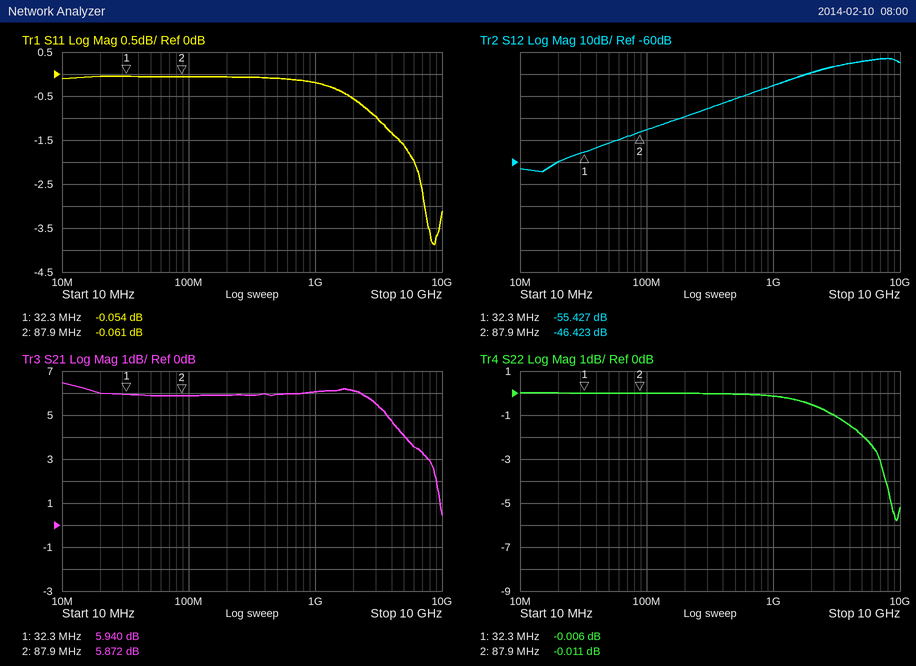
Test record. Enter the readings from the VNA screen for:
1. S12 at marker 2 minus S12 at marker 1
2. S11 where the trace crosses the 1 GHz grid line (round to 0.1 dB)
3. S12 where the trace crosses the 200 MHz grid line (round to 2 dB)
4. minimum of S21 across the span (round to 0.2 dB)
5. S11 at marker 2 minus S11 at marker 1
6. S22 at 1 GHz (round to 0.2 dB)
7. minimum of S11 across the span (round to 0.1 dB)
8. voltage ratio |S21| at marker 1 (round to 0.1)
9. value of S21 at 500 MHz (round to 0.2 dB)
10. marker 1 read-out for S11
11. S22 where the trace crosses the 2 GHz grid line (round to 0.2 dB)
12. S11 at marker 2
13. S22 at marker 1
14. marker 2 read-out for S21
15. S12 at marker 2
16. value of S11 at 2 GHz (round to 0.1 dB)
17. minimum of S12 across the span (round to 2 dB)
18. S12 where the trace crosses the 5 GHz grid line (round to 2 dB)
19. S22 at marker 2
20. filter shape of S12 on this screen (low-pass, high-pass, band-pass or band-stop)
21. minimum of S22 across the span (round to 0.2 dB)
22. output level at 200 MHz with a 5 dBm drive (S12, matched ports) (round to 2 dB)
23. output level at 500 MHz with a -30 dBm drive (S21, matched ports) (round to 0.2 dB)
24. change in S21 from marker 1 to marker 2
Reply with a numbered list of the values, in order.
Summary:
1. 9.004 dB
2. -0.2 dB
3. -40 dB
4. 0.4 dB
5. -0.007 dB
6. -0.2 dB
7. -3.9 dB
8. 2.0
9. 6.0 dB
10. -0.054 dB
11. -0.6 dB
12. -0.061 dB
13. -0.006 dB
14. 5.872 dB
15. -46.423 dB
16. -0.6 dB
17. -64 dB
18. -14 dB
19. -0.011 dB
20. high-pass
21. -5.8 dB
22. -34 dBm
23. -24.0 dBm
24. -0.068 dB
